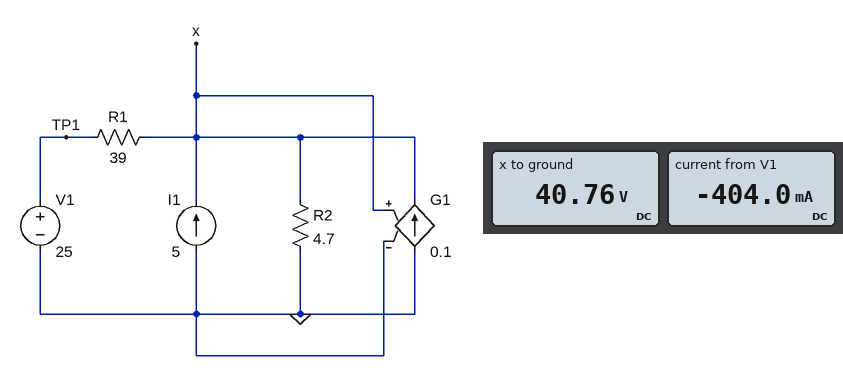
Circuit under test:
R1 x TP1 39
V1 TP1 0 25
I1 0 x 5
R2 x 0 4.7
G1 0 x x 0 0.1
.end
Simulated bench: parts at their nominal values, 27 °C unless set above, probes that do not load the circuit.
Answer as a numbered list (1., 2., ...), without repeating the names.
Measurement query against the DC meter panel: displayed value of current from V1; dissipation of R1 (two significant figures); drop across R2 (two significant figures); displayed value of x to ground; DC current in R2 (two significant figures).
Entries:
1. -404.0 mA
2. 6.4 W
3. 41 V
4. 40.76 V
5. 8.7 A
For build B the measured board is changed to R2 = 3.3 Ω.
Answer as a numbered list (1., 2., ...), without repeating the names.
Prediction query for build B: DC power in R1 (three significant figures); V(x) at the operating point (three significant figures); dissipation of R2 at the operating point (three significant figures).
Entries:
1. 2.81 mW
2. 24.7 V
3. 184 W
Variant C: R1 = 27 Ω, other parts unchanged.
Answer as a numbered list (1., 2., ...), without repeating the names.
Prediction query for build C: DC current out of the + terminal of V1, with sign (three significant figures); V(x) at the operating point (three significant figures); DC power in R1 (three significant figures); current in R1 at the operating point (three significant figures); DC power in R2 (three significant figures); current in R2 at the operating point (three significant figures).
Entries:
1. -539 mA
2. 39.6 V
3. 7.85 W
4. 539 mA
5. 333 W
6. 8.42 A
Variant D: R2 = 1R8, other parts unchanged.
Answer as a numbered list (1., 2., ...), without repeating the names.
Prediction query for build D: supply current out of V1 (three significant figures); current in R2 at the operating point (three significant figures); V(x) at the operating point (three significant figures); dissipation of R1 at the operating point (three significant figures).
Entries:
1. 340 mA
2. 6.51 A
3. 11.7 V
4. 4.52 W
